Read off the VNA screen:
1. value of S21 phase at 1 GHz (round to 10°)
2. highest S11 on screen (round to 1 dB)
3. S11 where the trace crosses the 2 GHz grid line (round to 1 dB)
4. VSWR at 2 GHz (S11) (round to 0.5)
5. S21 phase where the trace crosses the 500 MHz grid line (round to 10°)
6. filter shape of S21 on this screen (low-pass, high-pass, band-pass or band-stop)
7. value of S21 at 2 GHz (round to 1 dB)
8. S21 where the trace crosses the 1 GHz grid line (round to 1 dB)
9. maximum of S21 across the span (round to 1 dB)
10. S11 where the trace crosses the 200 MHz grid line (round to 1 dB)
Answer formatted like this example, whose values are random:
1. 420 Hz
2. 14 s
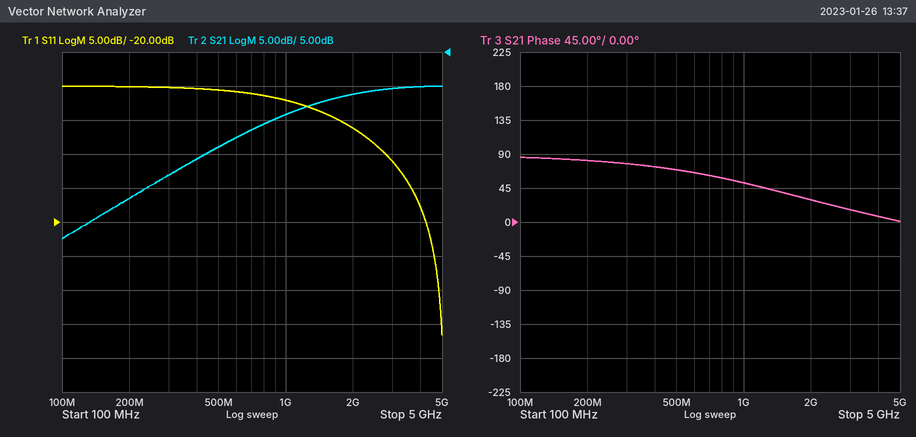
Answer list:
1. 50°
2. 0 dB
3. -6 dB
4. 3.0
5. 70°
6. high-pass
7. -1 dB
8. -4 dB
9. 0 dB
10. 0 dB
